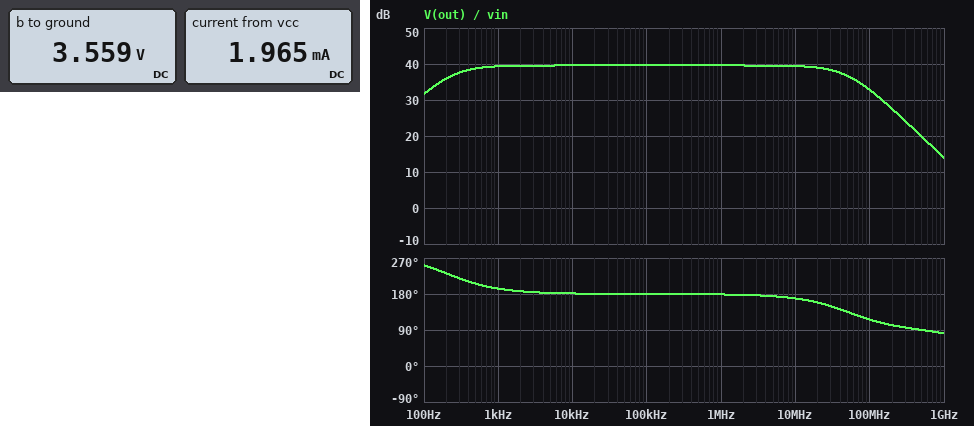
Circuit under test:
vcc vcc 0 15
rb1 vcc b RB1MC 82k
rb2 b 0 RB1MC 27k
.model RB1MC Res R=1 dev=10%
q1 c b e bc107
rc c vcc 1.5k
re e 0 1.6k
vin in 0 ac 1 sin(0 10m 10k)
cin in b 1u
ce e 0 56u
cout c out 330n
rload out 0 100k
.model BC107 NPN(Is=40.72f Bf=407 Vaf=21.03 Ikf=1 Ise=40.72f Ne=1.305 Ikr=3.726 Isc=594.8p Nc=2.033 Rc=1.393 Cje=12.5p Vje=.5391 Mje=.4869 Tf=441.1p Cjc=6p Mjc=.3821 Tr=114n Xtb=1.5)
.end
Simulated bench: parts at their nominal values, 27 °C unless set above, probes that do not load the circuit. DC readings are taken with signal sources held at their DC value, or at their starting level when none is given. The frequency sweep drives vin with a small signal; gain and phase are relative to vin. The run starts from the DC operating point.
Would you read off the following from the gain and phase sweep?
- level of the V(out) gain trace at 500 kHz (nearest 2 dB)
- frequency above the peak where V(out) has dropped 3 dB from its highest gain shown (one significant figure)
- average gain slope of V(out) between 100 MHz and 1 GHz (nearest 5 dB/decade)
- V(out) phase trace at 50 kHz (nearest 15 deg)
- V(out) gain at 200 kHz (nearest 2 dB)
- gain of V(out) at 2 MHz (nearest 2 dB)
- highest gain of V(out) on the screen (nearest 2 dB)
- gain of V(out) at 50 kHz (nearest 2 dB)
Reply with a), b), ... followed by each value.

a) 40 dB
b) 50 MHz
c) -20 dB/decade
d) 180 deg
e) 40 dB
f) 40 dB
g) 40 dB
h) 40 dB
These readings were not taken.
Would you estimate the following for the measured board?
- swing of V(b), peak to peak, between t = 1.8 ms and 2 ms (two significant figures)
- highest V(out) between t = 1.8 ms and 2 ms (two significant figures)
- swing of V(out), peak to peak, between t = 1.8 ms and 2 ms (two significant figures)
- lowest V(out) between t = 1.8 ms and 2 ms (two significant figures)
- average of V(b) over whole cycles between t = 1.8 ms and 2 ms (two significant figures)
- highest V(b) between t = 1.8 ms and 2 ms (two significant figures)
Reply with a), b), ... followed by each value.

a) 20 mV
b) 870 mV
c) 1.9 V
d) -1.0 V
e) 3.6 V
f) 3.6 V
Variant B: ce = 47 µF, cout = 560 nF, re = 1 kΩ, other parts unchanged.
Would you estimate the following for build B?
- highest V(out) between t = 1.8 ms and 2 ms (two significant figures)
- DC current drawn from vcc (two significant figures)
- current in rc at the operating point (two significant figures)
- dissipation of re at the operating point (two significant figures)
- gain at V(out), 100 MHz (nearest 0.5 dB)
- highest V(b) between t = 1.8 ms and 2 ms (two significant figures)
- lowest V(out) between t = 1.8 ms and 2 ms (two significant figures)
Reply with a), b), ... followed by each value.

a) 1.3 V
b) 3.0 mA
c) 2.8 mA
d) 8.1 mW
e) 36.0 dB
f) 3.5 V
g) -1.5 V
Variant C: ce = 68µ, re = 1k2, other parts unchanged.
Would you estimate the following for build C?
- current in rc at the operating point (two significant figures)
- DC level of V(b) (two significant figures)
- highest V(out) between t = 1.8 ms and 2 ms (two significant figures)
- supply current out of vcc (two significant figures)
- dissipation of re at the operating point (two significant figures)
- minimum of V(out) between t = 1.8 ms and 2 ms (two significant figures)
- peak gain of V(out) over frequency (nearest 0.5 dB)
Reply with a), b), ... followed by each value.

a) 2.4 mA
b) 3.5 V
c) 1.1 V
d) 2.5 mA
e) 6.9 mW
f) -1.3 V
g) 41.5 dB
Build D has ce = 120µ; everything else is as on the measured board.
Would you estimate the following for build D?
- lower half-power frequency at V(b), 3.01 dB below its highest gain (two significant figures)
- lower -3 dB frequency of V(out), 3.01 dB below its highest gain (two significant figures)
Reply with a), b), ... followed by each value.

a) 46 Hz
b) 130 Hz
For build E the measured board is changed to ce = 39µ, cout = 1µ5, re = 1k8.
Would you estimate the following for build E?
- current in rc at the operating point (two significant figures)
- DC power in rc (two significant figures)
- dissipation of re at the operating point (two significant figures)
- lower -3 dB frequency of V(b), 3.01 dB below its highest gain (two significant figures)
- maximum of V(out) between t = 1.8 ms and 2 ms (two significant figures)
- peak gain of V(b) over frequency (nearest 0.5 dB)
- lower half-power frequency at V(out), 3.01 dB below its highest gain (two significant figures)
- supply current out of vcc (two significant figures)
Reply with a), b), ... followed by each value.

a) 1.6 mA
b) 4.0 mW
c) 4.8 mW
d) 10 Hz
e) 780 mV
f) 0 dB
g) 280 Hz
h) 1.8 mA
